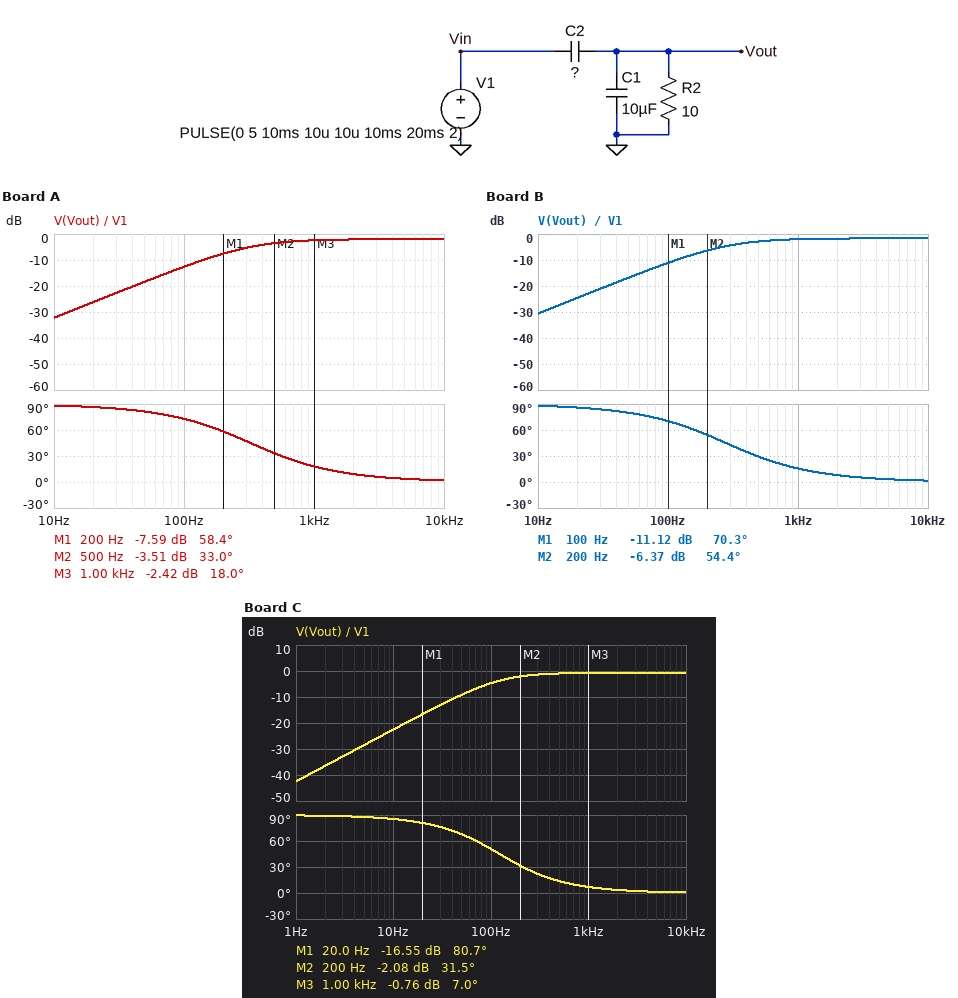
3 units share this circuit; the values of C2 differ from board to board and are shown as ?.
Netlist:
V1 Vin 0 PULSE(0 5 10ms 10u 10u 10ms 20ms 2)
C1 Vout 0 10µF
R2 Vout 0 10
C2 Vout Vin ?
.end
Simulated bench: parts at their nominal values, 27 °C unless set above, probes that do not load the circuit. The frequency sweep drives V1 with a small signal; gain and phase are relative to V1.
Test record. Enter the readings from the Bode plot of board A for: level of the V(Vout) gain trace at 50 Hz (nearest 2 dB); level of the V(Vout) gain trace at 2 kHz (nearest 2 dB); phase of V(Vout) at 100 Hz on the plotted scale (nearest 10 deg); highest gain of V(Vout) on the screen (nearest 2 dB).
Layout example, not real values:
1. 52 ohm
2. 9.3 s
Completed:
1. -18 dB
2. -2 dB
3. 70 deg
4. -2 dB
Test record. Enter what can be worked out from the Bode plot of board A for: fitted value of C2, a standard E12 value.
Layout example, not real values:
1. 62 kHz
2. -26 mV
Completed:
1. 39 µF
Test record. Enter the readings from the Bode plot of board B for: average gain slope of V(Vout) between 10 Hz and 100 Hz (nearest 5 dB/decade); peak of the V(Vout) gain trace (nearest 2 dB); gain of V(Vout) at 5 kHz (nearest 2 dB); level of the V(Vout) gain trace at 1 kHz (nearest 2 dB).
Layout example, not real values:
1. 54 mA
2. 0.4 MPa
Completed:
1. 20 dB/decade
2. -2 dB
3. -2 dB
4. -2 dB
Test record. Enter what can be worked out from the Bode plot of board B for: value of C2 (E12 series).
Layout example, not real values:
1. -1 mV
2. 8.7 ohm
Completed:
1. 47 µF
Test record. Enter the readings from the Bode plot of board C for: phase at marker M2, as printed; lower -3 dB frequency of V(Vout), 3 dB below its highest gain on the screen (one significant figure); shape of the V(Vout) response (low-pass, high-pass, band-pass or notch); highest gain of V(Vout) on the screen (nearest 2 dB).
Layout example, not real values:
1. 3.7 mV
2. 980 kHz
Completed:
1. 31.5 deg
2. 100 Hz
3. high-pass
4. 0 dB
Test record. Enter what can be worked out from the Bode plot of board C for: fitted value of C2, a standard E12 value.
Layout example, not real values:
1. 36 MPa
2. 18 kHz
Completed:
1. 120 µF
